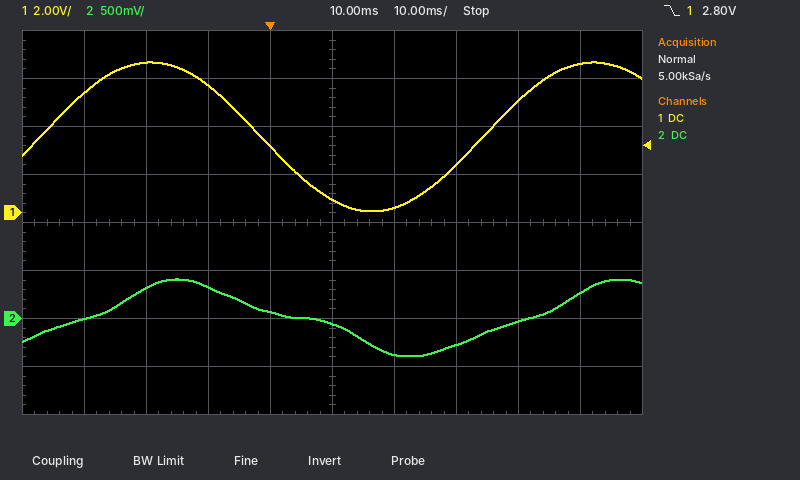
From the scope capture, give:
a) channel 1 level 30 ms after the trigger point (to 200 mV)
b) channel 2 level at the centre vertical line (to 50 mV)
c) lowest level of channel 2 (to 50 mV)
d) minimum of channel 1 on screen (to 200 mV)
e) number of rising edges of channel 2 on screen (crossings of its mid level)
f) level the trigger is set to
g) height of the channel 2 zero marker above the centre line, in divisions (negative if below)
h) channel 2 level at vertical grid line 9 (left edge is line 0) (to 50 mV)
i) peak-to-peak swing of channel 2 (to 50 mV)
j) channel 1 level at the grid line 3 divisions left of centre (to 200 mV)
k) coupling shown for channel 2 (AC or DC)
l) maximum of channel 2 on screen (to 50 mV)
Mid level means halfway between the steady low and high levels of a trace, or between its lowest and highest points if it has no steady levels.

2.0 V
-50 mV
-400 mV
0.0 V
2
2.80 V
-2.0 div
250 mV
800 mV
6.2 V
DC
400 mV
